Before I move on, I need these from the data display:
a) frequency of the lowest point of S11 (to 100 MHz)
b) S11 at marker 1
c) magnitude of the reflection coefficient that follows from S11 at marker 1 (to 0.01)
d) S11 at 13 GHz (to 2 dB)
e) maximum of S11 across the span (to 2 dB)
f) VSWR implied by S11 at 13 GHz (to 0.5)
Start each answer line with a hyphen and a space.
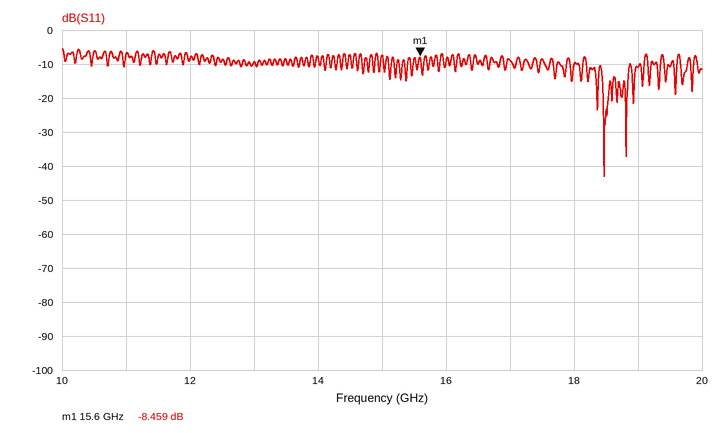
- 18.5 GHz
- -8.459 dB
- 0.38
- -10 dB
- -6 dB
- 2.0
